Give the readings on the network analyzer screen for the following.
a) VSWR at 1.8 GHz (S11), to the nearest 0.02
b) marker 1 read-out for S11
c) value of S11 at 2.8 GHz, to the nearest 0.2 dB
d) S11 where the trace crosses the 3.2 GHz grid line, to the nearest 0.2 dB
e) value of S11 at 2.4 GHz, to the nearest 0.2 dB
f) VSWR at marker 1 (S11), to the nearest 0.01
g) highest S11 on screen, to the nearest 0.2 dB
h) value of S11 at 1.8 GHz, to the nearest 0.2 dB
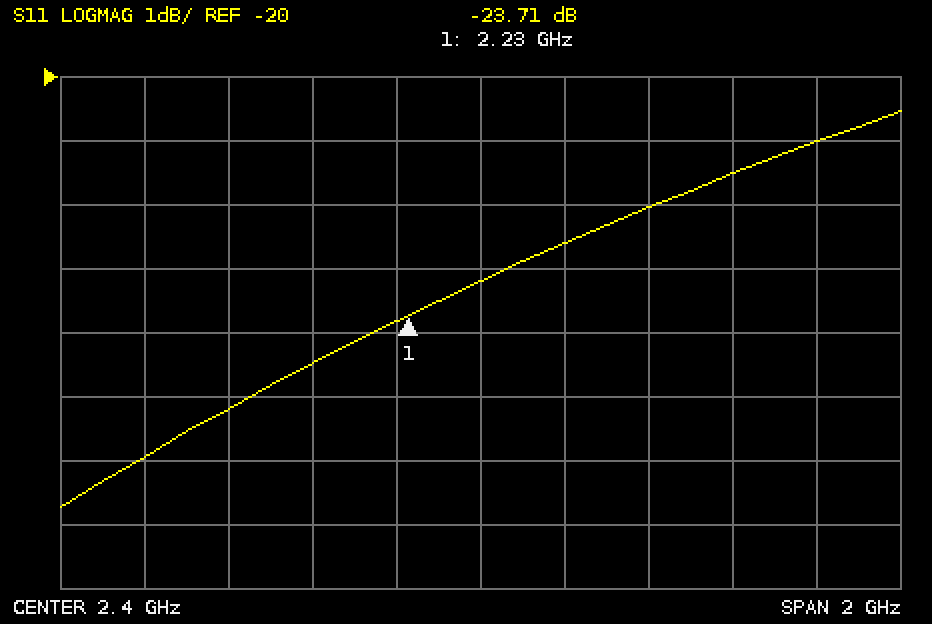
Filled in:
1.12
-23.71 dB
-22.0 dB
-21.0 dB
-23.2 dB
1.14
-20.6 dB
-25.2 dB
